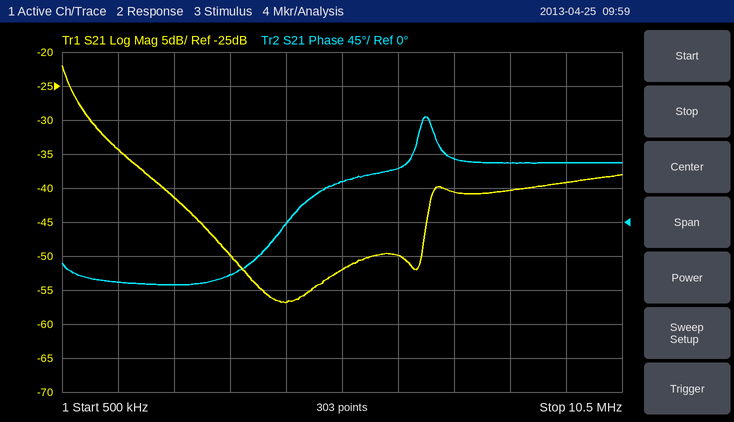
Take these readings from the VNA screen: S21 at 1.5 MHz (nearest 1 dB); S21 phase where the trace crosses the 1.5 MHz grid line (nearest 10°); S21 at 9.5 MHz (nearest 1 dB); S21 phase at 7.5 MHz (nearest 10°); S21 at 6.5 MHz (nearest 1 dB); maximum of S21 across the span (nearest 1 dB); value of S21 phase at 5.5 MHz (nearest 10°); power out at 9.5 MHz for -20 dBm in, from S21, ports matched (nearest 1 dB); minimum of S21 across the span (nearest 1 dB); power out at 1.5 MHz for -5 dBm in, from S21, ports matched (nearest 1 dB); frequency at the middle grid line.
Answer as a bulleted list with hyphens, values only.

- -34 dB
- -80°
- -39 dB
- 80°
- -50 dB
- -22 dB
- 50°
- -59 dBm
- -57 dB
- -39 dBm
- 5.5 MHz
